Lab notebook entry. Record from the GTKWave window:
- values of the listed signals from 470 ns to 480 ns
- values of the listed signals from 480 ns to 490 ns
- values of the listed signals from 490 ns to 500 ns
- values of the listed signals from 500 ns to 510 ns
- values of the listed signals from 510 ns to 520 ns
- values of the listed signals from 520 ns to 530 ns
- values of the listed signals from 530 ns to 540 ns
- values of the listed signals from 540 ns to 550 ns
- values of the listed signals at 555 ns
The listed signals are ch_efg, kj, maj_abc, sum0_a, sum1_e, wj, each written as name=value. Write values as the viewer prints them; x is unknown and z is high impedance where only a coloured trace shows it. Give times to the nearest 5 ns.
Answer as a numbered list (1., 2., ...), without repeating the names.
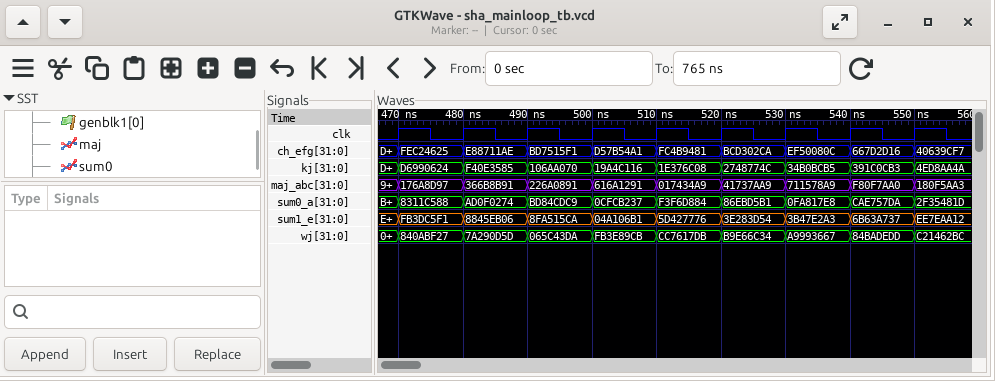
1. ch_efg=FEC24625, kj=D6990624, maj_abc=176A8D97, sum0_a=8311C588, sum1_e=FB3DC5F1, wj=840ABF27
2. ch_efg=E88711AE, kj=F40E3585, maj_abc=366B8B91, sum0_a=AD0F0274, sum1_e=8845EB06, wj=7A290D5D
3. ch_efg=BD7515F1, kj=106AA070, maj_abc=226A0891, sum0_a=BD84CDC9, sum1_e=8FA515CA, wj=065C43DA
4. ch_efg=D57B54A1, kj=19A4C116, maj_abc=616A1291, sum0_a=0CFCB237, sum1_e=04A106B1, wj=FB3E89CB
5. ch_efg=FC4B9481, kj=1E376C08, maj_abc=017434A9, sum0_a=F3F6D884, sum1_e=5D427776, wj=CC7617DB
6. ch_efg=BCD302CA, kj=2748774C, maj_abc=41737AA9, sum0_a=86EBD5B1, sum1_e=3E283D54, wj=B9E66C34
7. ch_efg=EF50080C, kj=34B0BCB5, maj_abc=711578A9, sum0_a=0FA817E8, sum1_e=3B47E2A3, wj=A9993667
8. ch_efg=667D2D16, kj=391C0CB3, maj_abc=F80F7AA0, sum0_a=CAE757DA, sum1_e=6B63A737, wj=84BADEDD
9. ch_efg=40639CF7, kj=4ED8AA4A, maj_abc=180F5AA3, sum0_a=2F35481D, sum1_e=EE7EAA12, wj=C21462BC
